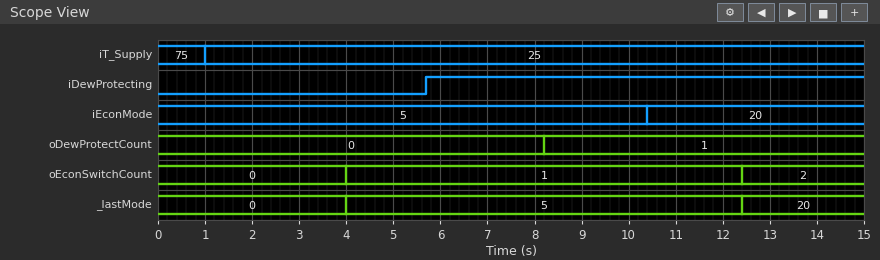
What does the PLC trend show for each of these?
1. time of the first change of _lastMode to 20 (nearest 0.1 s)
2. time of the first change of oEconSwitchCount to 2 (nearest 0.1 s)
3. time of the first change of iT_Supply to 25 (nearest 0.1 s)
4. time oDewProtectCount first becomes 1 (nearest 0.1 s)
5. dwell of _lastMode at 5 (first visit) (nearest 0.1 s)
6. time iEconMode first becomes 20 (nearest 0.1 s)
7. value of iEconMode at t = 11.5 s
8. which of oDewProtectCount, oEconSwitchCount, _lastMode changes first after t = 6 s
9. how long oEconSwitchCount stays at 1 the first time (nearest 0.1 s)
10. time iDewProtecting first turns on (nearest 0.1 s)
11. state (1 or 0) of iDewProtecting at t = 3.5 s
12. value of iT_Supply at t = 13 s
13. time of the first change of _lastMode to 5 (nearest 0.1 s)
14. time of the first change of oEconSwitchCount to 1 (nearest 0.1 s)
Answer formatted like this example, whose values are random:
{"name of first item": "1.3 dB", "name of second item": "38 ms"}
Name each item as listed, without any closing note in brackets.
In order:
{"time of the first change of _lastMode to 20": "12.4 s", "time of the first change of oEconSwitchCount to 2": "12.4 s", "time of the first change of iT_Supply to 25": "1.0 s", "time oDewProtectCount first becomes 1": "8.2 s", "dwell of _lastMode at 5 (first visit)": "8.4 s", "time iEconMode first becomes 20": "10.4 s", "value of iEconMode at t = 11.5 s": "20", "which of oDewProtectCount, oEconSwitchCount, _lastMode changes first after t = 6 s": "oDewProtectCount", "how long oEconSwitchCount stays at 1 the first time": "8.4 s", "time iDewProtecting first turns on": "5.7 s", "state (1 or 0) of iDewProtecting at t = 3.5 s": "0", "value of iT_Supply at t = 13 s": "25", "time of the first change of _lastMode to 5": "4.0 s", "time of the first change of oEconSwitchCount to 1": "4.0 s"}
